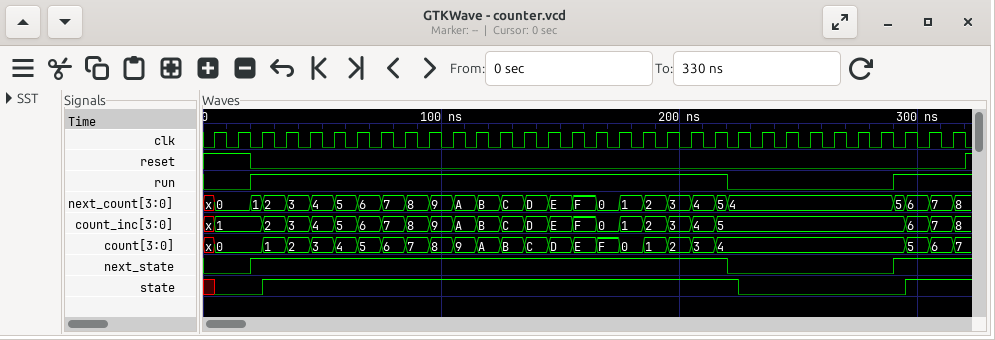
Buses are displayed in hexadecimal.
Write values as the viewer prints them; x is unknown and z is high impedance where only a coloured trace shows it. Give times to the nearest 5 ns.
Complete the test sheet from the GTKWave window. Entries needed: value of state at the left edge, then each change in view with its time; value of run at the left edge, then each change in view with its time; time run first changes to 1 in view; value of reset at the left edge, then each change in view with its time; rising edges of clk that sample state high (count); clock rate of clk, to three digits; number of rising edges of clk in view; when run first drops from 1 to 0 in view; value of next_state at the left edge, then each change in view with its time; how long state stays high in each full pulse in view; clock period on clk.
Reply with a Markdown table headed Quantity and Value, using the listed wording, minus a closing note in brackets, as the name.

| Quantity | Value |
|---|---|
| value of state at the left edge, then each change in view with its time | x, 0 at 5 ns, 1 at 25 ns, 0 at 225 ns, 1 at 295 ns |
| value of run at the left edge, then each change in view with its time | 0, 1 at 20 ns, 0 at 220 ns, 1 at 290 ns |
| time run first changes to 1 in view | 20 ns |
| value of reset at the left edge, then each change in view with its time | 1, 0 at 20 ns, 1 at 320 ns |
| rising edges of clk that sample state high | 22 |
| clock rate of clk, to three digits | 100 MHz |
| number of rising edges of clk in view | 32 |
| when run first drops from 1 to 0 in view | 220 ns |
| value of next_state at the left edge, then each change in view with its time | 0, 1 at 20 ns, 0 at 220 ns, 1 at 290 ns |
| how long state stays high in each full pulse in view | 200 ns |
| clock period on clk | 10 ns |
